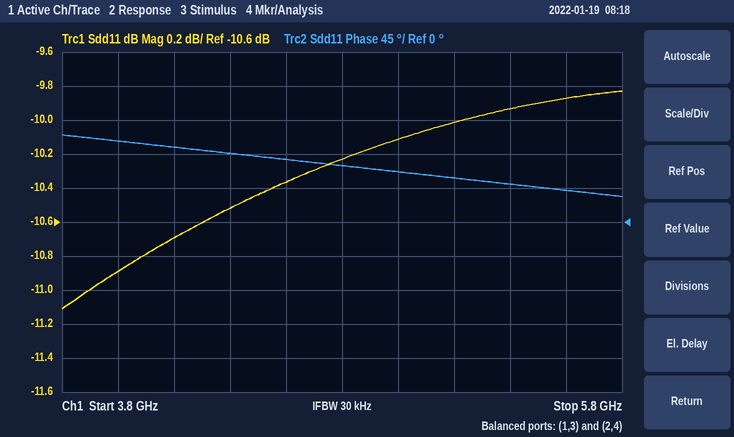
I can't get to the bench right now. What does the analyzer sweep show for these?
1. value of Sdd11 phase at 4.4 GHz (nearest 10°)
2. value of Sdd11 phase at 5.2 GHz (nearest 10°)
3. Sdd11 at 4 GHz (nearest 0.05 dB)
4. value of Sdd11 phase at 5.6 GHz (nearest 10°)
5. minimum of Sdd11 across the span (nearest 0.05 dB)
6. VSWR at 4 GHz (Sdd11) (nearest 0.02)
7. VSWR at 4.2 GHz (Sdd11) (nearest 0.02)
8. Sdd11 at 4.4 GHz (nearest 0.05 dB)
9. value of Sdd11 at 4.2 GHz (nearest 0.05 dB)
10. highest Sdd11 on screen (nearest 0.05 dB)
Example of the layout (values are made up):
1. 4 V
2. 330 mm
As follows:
1. 90°
2. 60°
3. -10.90 dB
4. 40°
5. -11.10 dB
6. 1.80
7. 1.82
8. -10.50 dB
9. -10.70 dB
10. -9.85 dB
